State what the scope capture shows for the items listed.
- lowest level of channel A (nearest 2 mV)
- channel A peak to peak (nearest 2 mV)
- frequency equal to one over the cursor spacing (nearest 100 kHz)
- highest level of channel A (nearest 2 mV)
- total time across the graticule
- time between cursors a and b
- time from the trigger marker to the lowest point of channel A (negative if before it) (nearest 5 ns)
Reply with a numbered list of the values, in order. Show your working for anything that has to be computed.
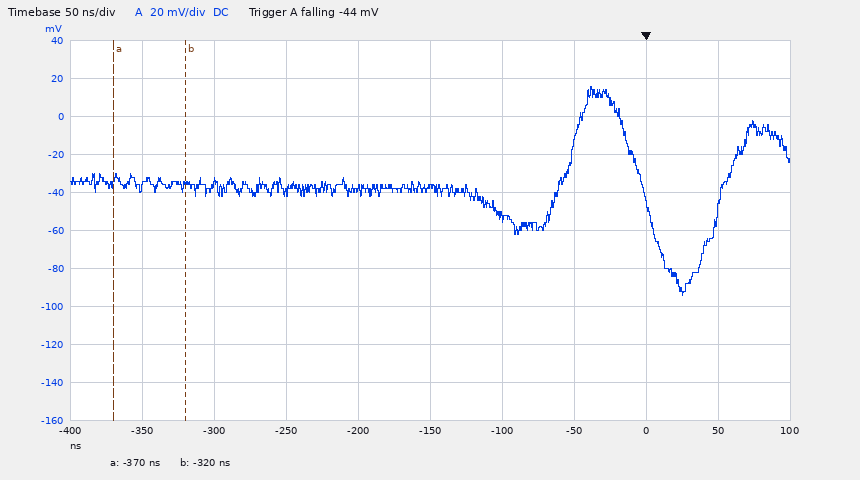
1. -94 mV
2. 16 mV − (-94 mV) = 110 mV
3. 1 / 50 ns ≈ 20.0 MHz
4. 16 mV
5. 500 ns
6. -320 ns − (-370 ns) = 50 ns
7. +25 ns
